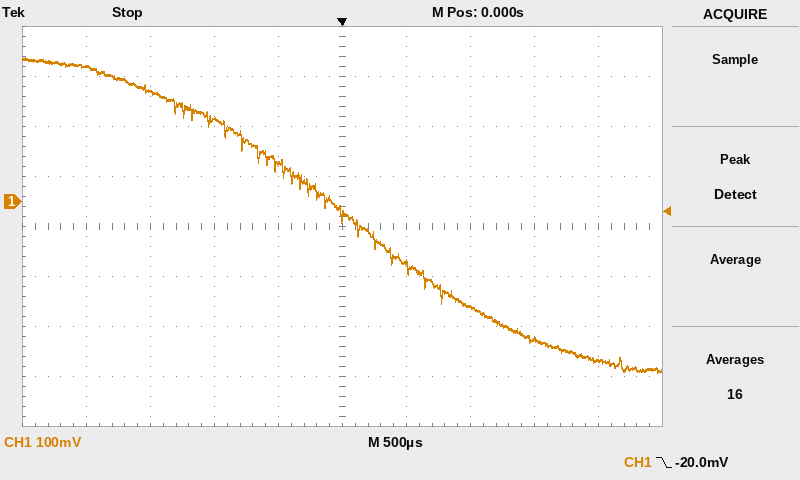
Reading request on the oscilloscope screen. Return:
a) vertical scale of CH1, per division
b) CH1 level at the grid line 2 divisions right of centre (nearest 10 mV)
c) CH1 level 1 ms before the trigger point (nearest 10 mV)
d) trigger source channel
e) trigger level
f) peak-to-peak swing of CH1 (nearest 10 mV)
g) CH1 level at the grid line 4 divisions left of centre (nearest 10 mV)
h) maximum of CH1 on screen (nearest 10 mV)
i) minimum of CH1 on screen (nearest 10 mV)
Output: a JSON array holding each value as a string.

["100 mV", "-210 mV", "160 mV", "CH1", "-20.0 mV", "630 mV", "270 mV", "290 mV", "-340 mV"]
